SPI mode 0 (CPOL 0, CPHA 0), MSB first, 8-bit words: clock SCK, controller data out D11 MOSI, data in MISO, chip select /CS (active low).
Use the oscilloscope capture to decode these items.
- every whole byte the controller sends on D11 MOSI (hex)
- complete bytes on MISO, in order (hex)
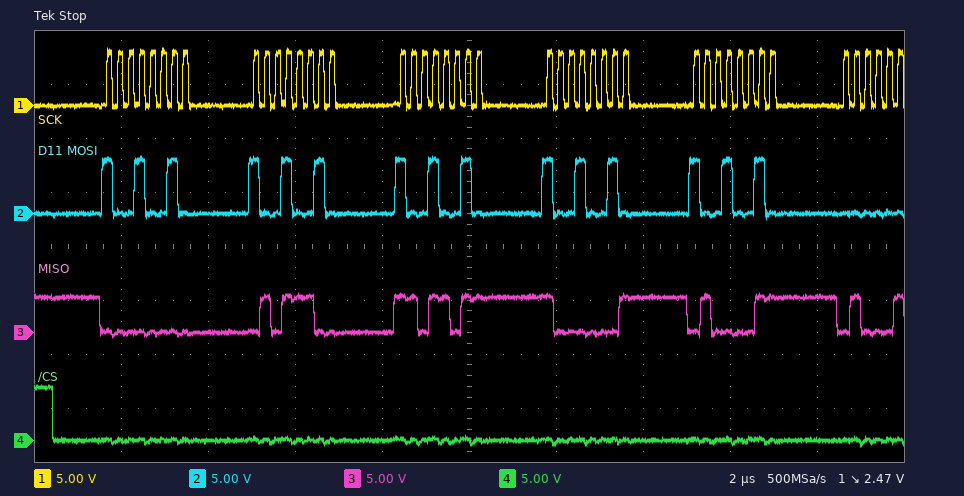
92 92 92 92 92
00 5C DB 81 43
